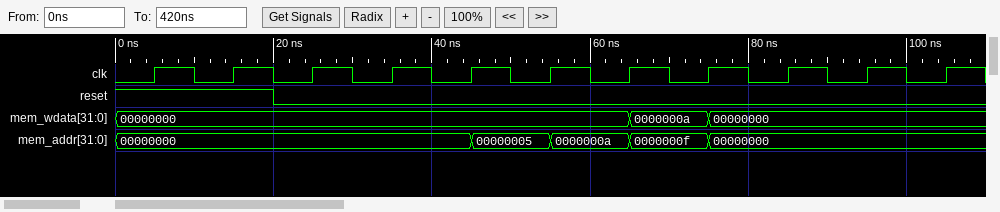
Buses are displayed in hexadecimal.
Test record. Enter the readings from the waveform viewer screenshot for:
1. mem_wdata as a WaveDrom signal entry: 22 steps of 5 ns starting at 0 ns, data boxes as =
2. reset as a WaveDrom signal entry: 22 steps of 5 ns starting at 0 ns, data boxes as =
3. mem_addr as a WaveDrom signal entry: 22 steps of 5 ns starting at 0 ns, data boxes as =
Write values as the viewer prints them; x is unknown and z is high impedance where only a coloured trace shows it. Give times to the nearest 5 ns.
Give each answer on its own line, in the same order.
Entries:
{name: 'mem_wdata', wave: '=............=.=......', data: '00000000 0000000a 00000000'}
{name: 'reset', wave: '1...0.................'}
{name: 'mem_addr', wave: '=........=.=.=.=......', data: '00000000 00000005 0000000a 0000000f 00000000'}
